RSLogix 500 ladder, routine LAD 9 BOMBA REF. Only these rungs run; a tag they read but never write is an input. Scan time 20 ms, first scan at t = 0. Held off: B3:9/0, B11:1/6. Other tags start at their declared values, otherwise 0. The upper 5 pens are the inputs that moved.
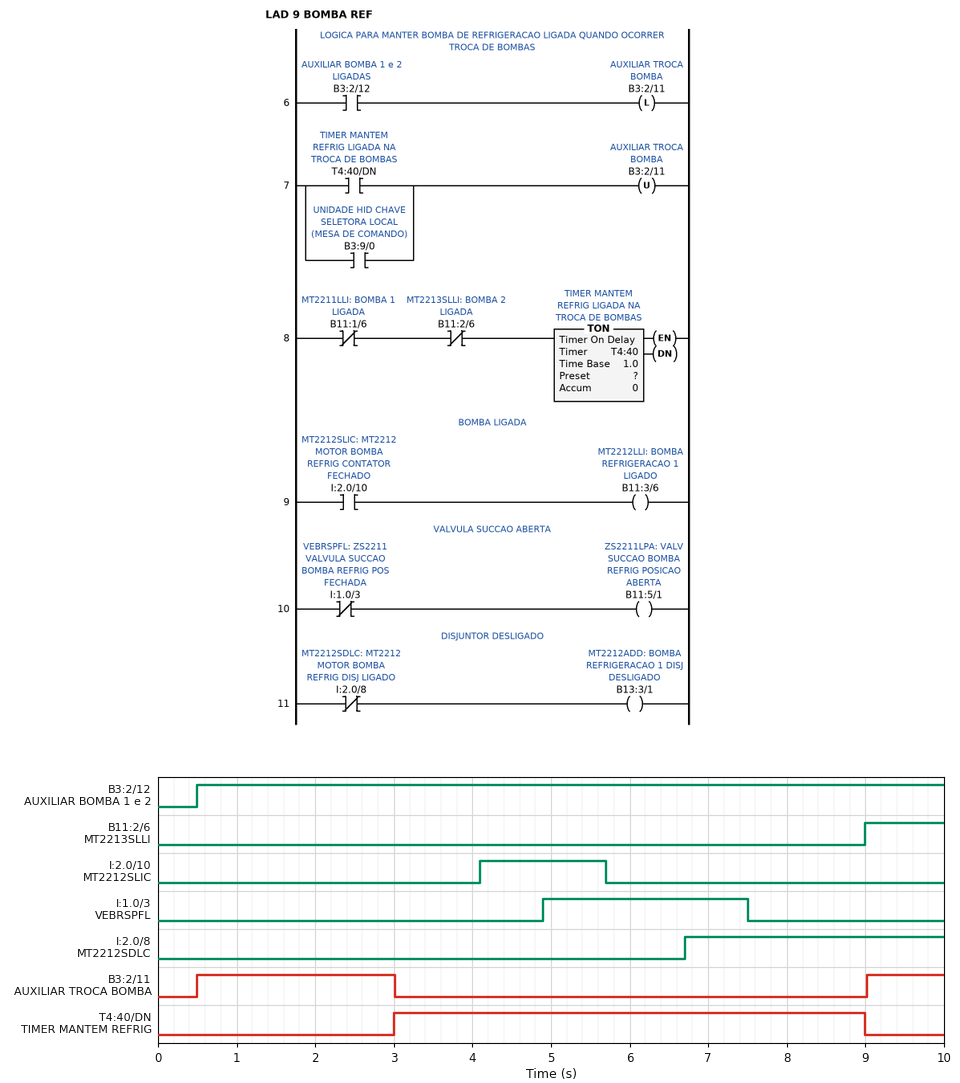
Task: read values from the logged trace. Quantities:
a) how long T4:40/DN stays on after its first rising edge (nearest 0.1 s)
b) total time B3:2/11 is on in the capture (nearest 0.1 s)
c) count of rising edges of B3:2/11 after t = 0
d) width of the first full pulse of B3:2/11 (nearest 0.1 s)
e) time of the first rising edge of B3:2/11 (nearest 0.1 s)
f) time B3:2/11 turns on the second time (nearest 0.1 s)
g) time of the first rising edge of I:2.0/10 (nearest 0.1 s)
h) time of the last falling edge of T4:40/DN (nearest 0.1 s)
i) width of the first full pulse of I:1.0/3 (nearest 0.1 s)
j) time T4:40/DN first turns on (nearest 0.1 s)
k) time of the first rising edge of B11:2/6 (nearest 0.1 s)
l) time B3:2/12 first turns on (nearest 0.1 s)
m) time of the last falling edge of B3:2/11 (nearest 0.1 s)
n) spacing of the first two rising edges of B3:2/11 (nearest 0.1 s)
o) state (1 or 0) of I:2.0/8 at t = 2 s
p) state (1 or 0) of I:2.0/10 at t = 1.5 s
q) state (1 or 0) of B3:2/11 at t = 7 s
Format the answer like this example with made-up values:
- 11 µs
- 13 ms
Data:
- 6.0 s
- 3.5 s
- 2
- 2.5 s
- 0.5 s
- 9.0 s
- 4.1 s
- 9.0 s
- 2.6 s
- 3.0 s
- 9.0 s
- 0.5 s
- 3.0 s
- 8.5 s
- 0
- 0
- 0
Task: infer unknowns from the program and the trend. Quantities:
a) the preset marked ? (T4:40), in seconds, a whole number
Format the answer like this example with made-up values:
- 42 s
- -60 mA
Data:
- 3 s
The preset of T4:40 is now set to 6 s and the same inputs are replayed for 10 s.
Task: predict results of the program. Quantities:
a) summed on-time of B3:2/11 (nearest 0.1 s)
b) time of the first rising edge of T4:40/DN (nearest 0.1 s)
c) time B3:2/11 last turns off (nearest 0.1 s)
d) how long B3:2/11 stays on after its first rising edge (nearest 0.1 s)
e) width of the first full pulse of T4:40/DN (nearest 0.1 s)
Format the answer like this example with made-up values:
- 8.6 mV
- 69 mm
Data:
- 6.5 s
- 6.0 s
- 6.0 s
- 5.5 s
- 3.0 s
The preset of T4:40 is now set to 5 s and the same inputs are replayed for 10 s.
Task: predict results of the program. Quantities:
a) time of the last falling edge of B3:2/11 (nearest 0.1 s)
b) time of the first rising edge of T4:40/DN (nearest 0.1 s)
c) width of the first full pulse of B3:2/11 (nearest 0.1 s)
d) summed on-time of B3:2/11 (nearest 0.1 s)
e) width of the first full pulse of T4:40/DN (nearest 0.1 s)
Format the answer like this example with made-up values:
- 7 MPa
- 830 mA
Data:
- 5.0 s
- 5.0 s
- 4.5 s
- 5.5 s
- 4.0 s
